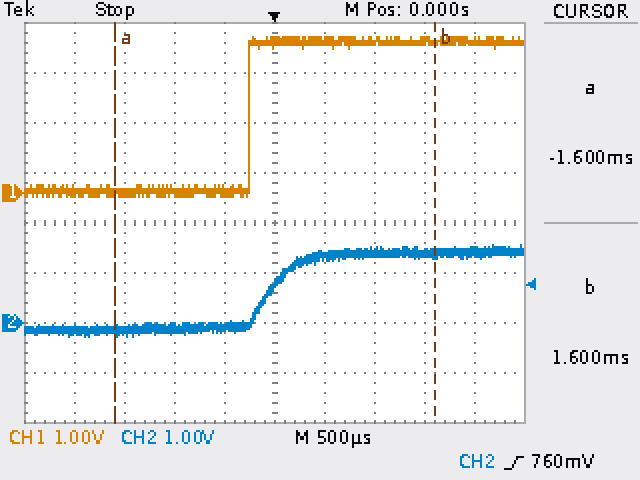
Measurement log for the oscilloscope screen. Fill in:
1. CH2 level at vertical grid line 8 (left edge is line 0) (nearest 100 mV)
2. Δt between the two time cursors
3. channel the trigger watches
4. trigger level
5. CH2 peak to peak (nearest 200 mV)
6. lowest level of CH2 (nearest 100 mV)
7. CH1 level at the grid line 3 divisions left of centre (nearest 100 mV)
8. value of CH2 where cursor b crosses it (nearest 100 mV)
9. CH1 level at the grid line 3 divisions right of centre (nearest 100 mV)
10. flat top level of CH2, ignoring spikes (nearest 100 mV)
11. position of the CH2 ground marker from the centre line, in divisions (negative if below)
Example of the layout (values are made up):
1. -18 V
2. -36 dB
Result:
1. 1.4 V
2. 3.20 ms
3. CH2
4. 760 mV
5. 1.8 V
6. -300 mV
7. 0.0 V
8. 1.4 V
9. 3.0 V
10. 1.4 V
11. -2.0 div
